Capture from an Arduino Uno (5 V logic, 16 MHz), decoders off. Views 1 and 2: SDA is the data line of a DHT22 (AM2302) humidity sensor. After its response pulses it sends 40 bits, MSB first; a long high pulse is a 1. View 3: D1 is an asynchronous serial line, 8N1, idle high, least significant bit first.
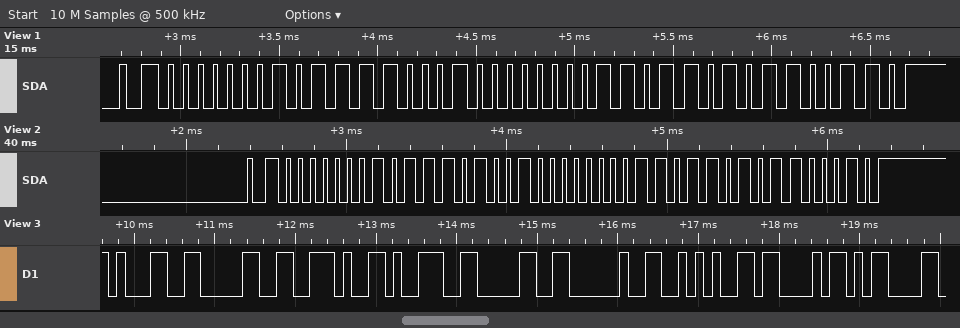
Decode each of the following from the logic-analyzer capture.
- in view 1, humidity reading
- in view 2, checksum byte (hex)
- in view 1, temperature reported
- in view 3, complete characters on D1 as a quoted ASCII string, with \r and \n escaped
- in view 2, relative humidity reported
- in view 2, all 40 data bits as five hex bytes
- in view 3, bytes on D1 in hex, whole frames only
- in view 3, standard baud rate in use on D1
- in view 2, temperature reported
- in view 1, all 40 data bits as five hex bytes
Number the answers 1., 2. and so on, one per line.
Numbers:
1. 37.6 %
2. 0x62
3. -10.9 °C
4. "10.90 *C\r"
5. 37.2 %
6. 01 74 80 6D 62
7. 31 30 2E 39 30 20 2A 43 0D
8. 9600 baud
9. -10.9 °C
10. 01 78 80 6D 66
